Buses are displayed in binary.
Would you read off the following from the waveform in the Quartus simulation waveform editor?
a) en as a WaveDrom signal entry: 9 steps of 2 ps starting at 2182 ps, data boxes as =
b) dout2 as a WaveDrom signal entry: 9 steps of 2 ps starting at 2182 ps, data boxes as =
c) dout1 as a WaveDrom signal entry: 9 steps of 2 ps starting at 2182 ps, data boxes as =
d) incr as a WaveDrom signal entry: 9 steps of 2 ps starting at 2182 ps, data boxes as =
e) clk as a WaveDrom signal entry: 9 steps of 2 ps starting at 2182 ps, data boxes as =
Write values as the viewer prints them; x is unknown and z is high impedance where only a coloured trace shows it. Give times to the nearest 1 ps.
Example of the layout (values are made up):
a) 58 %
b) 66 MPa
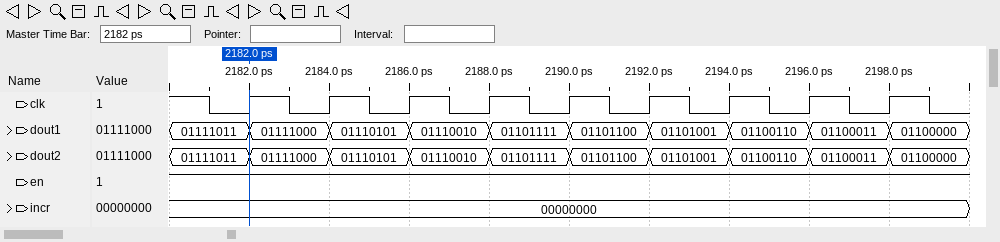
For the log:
a) {name: 'en', wave: '1........'}
b) {name: 'dout2', wave: '=========', data: '01111000 01110101 01110010 01101111 01101100 01101001 01100110 01100011 01100000'}
c) {name: 'dout1', wave: '=========', data: '01111000 01110101 01110010 01101111 01101100 01101001 01100110 01100011 01100000'}
d) {name: 'incr', wave: '=........', data: '00000000'}
e) {name: 'clk', wave: 'p........'}
